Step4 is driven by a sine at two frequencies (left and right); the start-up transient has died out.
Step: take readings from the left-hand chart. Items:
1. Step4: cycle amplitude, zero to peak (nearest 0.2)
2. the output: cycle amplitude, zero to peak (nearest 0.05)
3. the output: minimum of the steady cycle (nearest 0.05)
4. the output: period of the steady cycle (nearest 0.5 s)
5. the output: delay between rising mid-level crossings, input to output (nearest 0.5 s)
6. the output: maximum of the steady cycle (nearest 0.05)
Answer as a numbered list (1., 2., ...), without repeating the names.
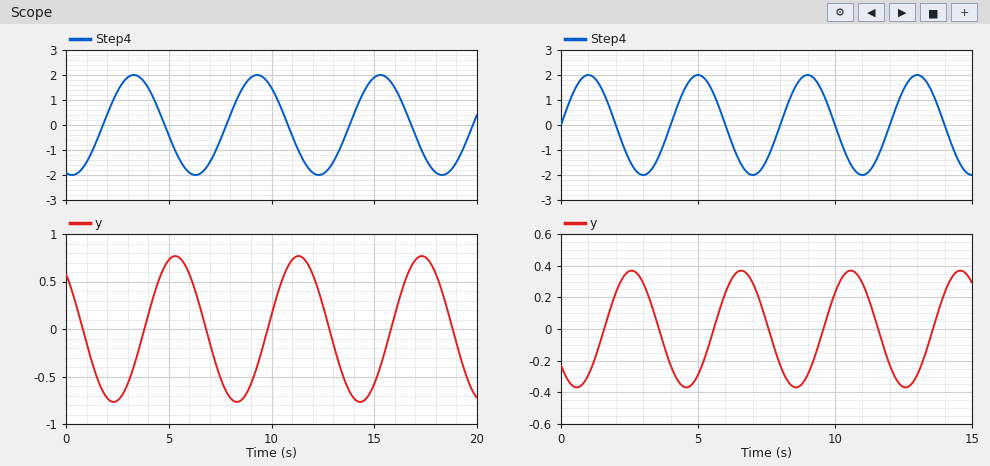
1. 2.0
2. 0.75
3. -0.75
4. 6.0 s
5. 2.0 s
6. 0.75
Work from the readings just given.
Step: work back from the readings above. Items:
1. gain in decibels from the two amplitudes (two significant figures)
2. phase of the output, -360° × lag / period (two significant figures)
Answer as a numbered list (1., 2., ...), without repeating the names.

1. -8.5 dB
2. -120°
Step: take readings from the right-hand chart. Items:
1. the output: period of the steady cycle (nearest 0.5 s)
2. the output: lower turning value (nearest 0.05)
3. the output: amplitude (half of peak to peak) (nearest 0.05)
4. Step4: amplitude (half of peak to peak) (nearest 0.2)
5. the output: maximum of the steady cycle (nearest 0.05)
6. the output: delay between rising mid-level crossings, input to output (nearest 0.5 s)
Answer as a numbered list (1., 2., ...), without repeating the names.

1. 4.0 s
2. -0.35
3. 0.35
4. 2.0
5. 0.35
6. 1.5 s
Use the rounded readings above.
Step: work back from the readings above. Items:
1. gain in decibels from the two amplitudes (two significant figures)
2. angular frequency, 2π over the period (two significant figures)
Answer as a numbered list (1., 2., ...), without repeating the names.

1. -15 dB
2. 1.6 rad/s
